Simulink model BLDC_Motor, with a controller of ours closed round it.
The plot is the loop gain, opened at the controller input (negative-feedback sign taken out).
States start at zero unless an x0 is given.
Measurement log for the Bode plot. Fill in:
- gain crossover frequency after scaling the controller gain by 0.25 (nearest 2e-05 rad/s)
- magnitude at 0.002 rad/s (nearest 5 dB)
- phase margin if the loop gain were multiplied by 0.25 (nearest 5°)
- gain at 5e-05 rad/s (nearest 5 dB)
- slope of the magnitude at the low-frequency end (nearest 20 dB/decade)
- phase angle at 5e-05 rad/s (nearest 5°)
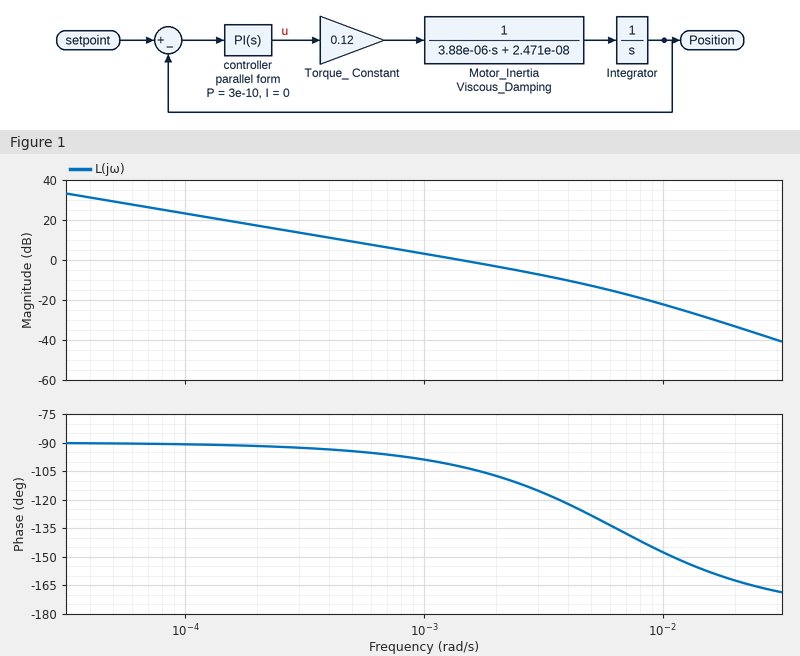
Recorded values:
0.00036 rad/s
-5 dB
85°
30 dB
-20 dB/decade
-90°
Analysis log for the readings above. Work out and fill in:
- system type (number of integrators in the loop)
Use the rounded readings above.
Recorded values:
1
